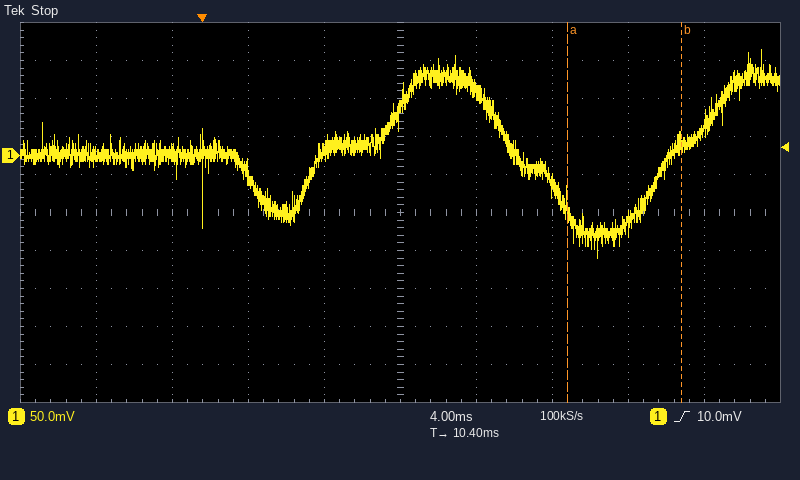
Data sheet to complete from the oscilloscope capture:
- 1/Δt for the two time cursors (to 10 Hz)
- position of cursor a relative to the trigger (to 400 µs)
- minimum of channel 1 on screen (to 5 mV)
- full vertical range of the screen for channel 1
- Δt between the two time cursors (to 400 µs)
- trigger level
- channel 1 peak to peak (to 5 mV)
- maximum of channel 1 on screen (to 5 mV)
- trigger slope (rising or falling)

170 Hz
+19.2 ms
-135 mV
500 mV
6.0 ms
10.0 mV
275 mV
140 mV
rising
